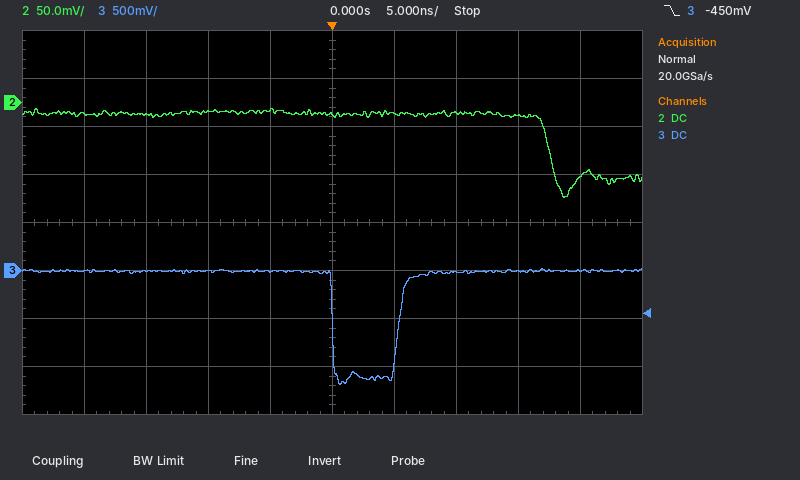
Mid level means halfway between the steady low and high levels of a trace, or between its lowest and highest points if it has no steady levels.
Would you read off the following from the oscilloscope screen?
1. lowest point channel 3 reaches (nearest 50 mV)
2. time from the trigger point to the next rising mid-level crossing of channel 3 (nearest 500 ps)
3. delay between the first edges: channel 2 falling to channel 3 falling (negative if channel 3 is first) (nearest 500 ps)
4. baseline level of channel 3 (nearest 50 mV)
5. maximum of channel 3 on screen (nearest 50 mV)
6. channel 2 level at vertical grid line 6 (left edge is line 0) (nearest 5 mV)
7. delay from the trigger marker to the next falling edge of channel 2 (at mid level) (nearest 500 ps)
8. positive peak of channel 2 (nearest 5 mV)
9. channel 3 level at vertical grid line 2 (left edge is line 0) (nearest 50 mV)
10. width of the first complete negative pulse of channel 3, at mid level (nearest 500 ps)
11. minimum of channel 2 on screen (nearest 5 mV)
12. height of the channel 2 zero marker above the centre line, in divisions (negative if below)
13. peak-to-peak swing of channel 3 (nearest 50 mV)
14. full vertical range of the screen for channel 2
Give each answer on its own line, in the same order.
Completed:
-1.20 V
5.5 ns
-17.5 ns
0 mV
0 mV
-10 mV
17.5 ns
-5 mV
0 mV
5.5 ns
-100 mV
+2.5 div
1.20 V
400 mV
